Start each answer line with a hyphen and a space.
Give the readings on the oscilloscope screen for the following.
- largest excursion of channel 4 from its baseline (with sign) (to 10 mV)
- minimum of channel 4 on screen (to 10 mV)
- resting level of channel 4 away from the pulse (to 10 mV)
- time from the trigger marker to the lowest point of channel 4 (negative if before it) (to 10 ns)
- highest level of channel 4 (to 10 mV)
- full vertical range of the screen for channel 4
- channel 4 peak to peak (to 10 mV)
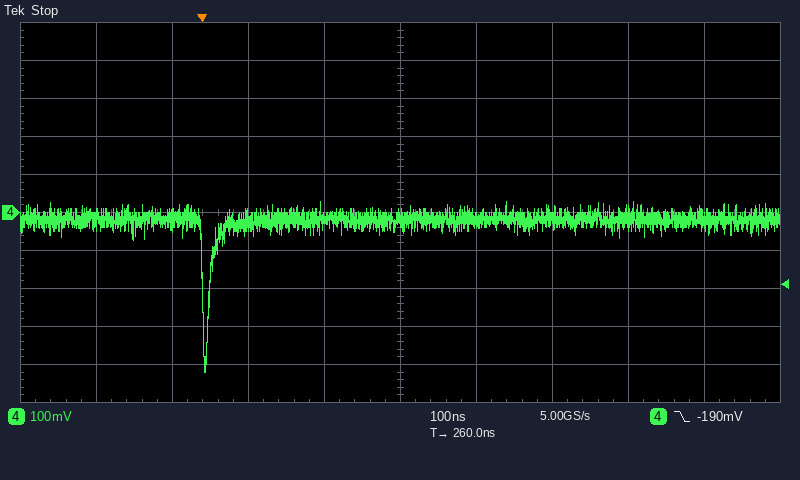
- -400 mV
- -420 mV
- -20 mV
- 0 ns
- 30 mV
- 1 V
- 450 mV
